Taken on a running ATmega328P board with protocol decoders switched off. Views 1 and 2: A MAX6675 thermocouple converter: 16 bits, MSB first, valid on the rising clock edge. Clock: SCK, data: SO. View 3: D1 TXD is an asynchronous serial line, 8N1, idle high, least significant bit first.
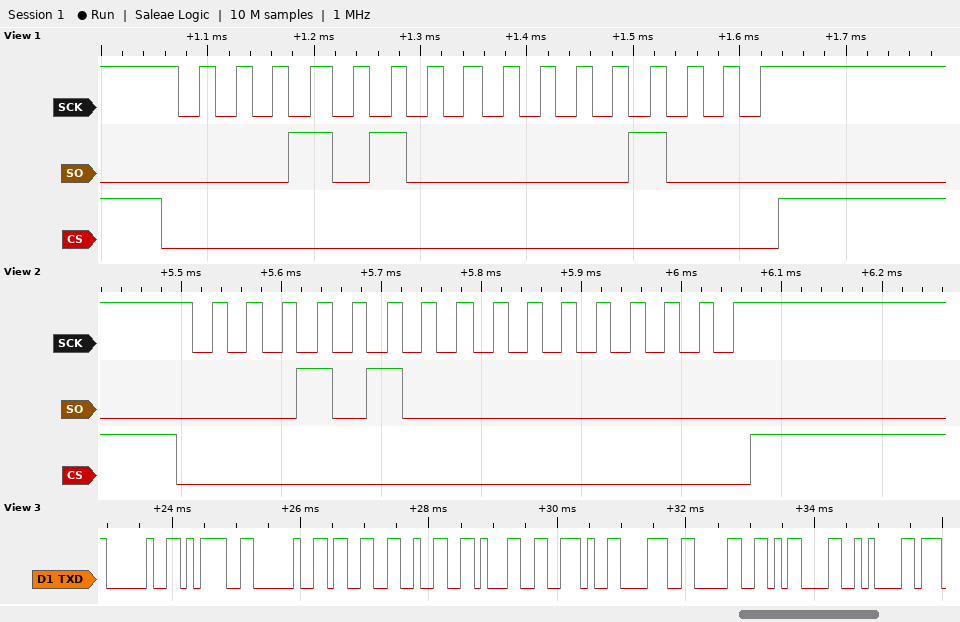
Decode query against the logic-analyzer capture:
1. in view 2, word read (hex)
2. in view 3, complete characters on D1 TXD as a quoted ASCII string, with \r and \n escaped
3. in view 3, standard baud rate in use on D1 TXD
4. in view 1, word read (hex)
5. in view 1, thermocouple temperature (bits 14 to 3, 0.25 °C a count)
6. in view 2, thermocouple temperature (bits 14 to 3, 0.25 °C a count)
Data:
0x1400
" = 321.80\r\n"
9600 baud
0x1408
160.25 °C
160.00 °C
